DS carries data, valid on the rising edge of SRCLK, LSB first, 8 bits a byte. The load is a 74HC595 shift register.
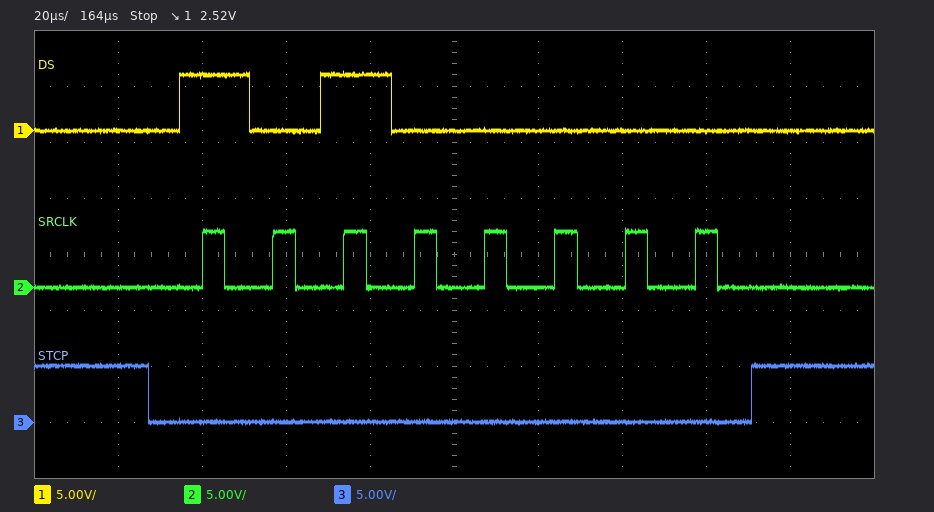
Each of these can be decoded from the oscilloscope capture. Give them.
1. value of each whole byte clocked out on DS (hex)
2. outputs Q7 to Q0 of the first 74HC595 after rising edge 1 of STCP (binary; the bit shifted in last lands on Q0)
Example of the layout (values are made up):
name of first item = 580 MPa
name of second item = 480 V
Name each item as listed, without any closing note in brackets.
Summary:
value of each whole byte clocked out on DS = 0x05
outputs Q7 to Q0 of the first 74HC595 after rising edge 1 of STCP = 10100000
